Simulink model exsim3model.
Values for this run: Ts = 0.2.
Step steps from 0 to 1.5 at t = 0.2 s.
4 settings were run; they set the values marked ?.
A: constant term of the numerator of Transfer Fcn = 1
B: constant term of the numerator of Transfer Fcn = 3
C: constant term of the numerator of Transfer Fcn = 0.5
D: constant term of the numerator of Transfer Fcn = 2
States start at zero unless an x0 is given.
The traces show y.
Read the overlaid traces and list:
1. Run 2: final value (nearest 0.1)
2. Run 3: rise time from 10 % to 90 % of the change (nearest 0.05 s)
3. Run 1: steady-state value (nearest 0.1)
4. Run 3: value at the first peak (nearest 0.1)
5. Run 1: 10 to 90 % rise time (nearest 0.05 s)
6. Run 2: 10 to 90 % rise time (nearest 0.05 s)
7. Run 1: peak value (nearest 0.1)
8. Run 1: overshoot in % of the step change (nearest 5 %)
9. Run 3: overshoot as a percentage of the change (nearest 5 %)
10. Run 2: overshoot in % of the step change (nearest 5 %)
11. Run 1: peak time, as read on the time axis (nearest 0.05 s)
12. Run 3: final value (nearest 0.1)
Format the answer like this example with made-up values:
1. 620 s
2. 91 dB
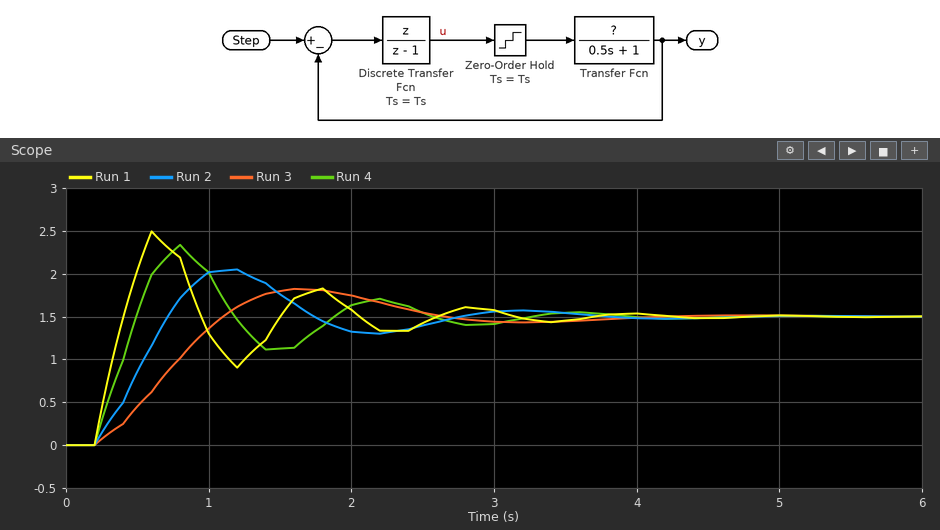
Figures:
1. 1.5
2. 0.70 s
3. 1.5
4. 1.8
5. 0.15 s
6. 0.40 s
7. 2.5
8. 65 %
9. 20 %
10. 35 %
11. 0.60 s
12. 1.5
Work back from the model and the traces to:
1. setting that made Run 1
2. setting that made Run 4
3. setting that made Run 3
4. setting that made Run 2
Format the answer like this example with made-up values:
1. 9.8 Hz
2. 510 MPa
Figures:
1. B
2. D
3. C
4. A
